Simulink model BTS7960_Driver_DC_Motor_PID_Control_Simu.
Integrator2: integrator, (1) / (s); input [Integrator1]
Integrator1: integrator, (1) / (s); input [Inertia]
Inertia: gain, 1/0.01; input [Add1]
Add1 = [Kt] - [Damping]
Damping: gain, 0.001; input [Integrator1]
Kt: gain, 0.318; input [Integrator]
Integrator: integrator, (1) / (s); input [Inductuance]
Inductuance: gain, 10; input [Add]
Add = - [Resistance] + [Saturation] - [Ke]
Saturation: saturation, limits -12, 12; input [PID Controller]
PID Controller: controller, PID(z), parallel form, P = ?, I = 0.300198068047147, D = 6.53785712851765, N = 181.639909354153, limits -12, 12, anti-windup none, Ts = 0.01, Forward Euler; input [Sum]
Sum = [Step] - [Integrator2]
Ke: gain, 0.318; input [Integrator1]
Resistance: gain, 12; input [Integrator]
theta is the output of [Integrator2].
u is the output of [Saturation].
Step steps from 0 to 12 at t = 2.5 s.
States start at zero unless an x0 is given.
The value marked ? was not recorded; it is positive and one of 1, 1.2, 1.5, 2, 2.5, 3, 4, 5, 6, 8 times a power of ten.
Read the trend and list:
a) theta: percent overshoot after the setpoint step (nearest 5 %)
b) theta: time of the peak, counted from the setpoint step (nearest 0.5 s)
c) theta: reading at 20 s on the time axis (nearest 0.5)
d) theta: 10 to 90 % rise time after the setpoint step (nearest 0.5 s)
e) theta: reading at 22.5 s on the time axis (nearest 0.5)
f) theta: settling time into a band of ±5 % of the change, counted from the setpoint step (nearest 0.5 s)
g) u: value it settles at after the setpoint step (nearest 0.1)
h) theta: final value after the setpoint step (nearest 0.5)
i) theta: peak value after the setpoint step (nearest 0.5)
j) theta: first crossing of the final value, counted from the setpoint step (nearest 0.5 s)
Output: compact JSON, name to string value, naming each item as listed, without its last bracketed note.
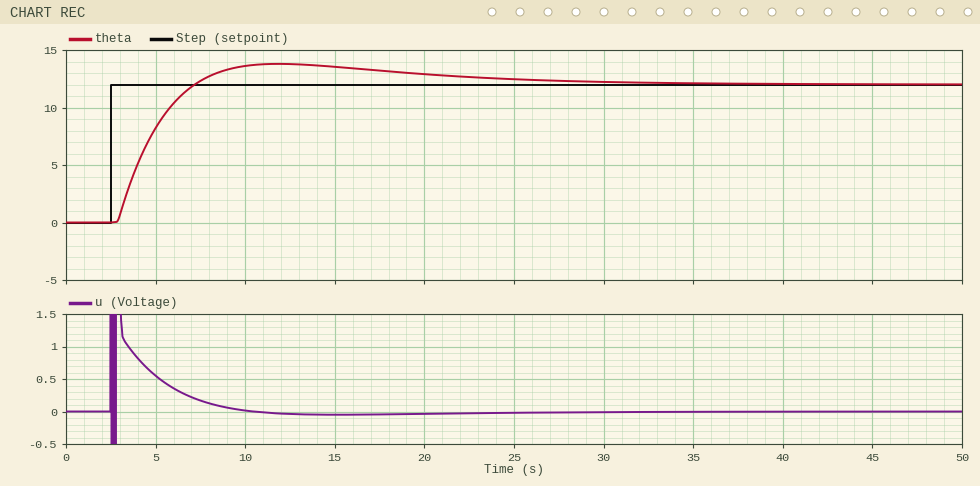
{"theta: percent overshoot after the setpoint step": "15 %", "theta: time of the peak, counted from the setpoint step": "9.5 s", "theta: reading at 20 s on the time axis": "13.0", "theta: 10 to 90 % rise time after the setpoint step": "3.0 s", "theta: reading at 22.5 s on the time axis": "12.5", "theta: settling time into a band of ±5 % of the change, counted from the setpoint step": "20.5 s", "u: value it settles at after the setpoint step": "0.0", "theta: final value after the setpoint step": "12.0", "theta: peak value after the setpoint step": "14.0", "theta: first crossing of the final value, counted from the setpoint step": "4.5 s"}
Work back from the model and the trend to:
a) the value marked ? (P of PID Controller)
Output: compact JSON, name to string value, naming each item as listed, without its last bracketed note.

{"the value marked ?": "3"}
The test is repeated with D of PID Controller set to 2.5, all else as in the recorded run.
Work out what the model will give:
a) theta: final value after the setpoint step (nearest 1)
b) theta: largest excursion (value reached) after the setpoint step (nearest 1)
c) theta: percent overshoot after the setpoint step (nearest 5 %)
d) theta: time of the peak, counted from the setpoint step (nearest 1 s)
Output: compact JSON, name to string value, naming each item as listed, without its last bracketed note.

{"theta: final value after the setpoint step": "12", "theta: largest excursion (value reached) after the setpoint step": "13", "theta: percent overshoot after the setpoint step": "10 %", "theta: time of the peak, counted from the setpoint step": "5 s"}
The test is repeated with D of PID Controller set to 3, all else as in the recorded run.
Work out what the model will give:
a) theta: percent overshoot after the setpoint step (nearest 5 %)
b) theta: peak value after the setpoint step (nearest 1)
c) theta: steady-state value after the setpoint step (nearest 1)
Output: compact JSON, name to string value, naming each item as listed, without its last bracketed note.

{"theta: percent overshoot after the setpoint step": "10 %", "theta: peak value after the setpoint step": "13", "theta: steady-state value after the setpoint step": "12"}
